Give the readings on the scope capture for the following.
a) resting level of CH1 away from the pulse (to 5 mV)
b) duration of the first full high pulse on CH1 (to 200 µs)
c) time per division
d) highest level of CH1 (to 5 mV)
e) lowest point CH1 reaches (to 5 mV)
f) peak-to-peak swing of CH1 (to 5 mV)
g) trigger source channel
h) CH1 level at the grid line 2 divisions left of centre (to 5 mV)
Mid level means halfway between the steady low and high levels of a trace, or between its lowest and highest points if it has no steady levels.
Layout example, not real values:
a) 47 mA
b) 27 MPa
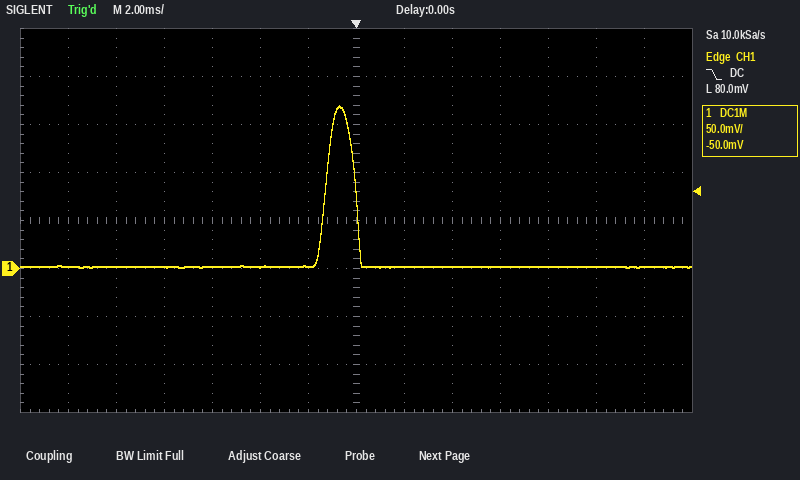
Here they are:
a) 0 mV
b) 1.2 ms
c) 2 ms
d) 170 mV
e) 0 mV
f) 170 mV
g) CH1
h) 0 mV
